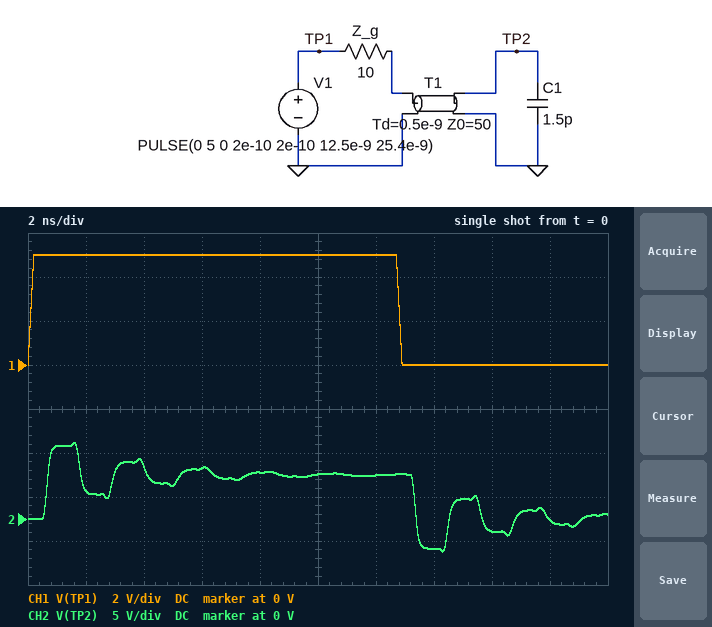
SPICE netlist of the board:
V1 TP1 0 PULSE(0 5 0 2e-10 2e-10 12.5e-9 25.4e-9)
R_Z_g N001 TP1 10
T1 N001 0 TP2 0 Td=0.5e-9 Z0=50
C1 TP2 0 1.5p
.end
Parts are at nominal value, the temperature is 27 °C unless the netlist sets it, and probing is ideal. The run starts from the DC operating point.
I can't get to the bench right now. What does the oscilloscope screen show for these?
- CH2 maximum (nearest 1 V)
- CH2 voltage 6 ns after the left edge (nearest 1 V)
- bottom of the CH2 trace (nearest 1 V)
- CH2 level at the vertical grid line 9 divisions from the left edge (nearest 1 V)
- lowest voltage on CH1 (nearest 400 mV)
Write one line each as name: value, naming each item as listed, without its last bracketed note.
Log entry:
CH2 maximum: 9 V
CH2 voltage 6 ns after the left edge: 6 V
bottom of the CH2 trace: -4 V
CH2 level at the vertical grid line 9 divisions from the left edge: 0 V
lowest voltage on CH1: 0 V
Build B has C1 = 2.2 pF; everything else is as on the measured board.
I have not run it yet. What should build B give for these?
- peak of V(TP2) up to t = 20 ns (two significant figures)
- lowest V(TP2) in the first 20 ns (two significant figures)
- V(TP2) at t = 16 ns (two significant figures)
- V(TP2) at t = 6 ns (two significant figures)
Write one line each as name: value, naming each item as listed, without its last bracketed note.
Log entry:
peak of V(TP2) up to t = 20 ns: 8.9 V
lowest V(TP2) in the first 20 ns: -3.9 V
V(TP2) at t = 16 ns: -900 mV
V(TP2) at t = 6 ns: 5.5 V
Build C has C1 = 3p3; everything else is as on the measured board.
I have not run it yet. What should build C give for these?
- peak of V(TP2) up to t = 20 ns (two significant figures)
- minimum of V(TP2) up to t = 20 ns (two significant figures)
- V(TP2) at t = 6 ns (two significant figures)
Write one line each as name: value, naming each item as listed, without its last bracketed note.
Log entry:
peak of V(TP2) up to t = 20 ns: 9.1 V
minimum of V(TP2) up to t = 20 ns: -4.1 V
V(TP2) at t = 6 ns: 5.0 V
